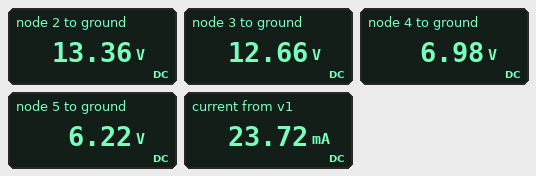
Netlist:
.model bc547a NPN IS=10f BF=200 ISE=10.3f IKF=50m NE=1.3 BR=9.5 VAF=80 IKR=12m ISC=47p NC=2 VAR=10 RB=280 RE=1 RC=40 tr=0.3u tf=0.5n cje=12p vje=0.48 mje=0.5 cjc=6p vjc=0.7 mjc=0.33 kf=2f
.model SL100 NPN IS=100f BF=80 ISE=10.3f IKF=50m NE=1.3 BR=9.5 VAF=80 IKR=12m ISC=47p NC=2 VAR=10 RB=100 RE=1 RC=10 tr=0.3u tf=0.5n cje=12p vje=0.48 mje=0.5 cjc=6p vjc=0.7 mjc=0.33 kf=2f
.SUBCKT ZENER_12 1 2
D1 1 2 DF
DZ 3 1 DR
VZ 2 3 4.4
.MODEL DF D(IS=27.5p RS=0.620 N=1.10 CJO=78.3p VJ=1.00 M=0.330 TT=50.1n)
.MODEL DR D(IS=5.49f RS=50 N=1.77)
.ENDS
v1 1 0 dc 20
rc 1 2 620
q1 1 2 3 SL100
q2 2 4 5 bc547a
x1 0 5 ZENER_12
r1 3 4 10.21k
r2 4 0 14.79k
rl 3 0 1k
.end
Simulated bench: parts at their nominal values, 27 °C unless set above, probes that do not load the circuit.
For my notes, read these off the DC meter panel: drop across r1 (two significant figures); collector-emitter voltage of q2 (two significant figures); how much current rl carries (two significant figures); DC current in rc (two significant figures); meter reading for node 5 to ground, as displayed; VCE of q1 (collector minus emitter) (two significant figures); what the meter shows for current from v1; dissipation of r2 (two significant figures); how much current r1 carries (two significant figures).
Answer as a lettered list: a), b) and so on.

a) 5.7 V
b) 7.1 V
c) 13 mA
d) 11 mA
e) 6.22 V
f) 7.3 V
g) 23.72 mA
h) 3.3 mW
i) 560 µA
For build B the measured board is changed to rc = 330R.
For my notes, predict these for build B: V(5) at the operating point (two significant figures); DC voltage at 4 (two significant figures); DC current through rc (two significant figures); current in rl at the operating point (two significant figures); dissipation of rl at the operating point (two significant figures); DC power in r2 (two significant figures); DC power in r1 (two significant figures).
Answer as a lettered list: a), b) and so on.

a) 6.5 V
b) 7.3 V
c) 17 mA
d) 14 mA
e) 190 mW
f) 3.6 mW
g) 4.1 mW
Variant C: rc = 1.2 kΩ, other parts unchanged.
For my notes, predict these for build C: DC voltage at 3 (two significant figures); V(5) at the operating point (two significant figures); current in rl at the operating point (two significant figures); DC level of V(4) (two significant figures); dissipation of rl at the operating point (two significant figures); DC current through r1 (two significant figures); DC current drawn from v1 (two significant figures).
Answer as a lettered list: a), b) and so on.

a) 12 V
b) 6.0 V
c) 12 mA
d) 6.7 V
e) 140 mW
f) 500 µA
g) 18 mA
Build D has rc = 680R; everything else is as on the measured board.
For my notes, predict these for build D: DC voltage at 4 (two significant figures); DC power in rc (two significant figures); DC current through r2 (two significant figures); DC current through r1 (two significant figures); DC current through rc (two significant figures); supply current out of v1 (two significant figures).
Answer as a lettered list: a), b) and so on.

a) 6.9 V
b) 68 mW
c) 470 µA
d) 550 µA
e) 10 mA
f) 23 mA
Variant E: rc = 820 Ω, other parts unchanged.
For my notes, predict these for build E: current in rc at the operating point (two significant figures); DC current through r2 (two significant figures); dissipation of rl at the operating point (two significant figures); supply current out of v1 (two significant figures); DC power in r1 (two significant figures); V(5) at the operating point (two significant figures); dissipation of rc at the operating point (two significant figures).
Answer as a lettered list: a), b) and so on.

a) 8.6 mA
b) 460 µA
c) 150 mW
d) 21 mA
e) 2.9 mW
f) 6.1 V
g) 61 mW
